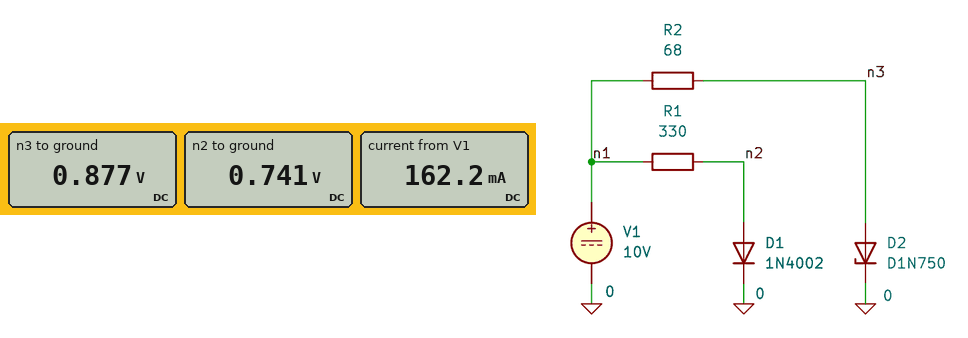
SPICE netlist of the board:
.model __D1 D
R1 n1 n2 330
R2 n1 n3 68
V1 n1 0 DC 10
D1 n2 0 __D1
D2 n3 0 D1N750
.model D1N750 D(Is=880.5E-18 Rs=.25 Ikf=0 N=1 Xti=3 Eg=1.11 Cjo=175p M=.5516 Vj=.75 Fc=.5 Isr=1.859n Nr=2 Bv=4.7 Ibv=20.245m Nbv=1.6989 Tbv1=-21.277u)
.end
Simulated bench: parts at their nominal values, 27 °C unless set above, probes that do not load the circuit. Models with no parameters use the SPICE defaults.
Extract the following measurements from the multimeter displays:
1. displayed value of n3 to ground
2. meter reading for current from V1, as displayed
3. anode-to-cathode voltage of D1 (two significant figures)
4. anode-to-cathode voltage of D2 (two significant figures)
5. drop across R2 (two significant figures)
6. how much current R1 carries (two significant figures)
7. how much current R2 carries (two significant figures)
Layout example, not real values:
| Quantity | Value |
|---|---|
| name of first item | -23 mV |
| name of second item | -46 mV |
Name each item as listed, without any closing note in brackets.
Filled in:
| Quantity | Value |
|---|---|
| displayed value of n3 to ground | 0.877 V |
| meter reading for current from V1, as displayed | 162.2 mA |
| anode-to-cathode voltage of D1 | 740 mV |
| anode-to-cathode voltage of D2 | 880 mV |
| drop across R2 | 9.1 V |
| how much current R1 carries | 28 mA |
| how much current R2 carries | 130 mA |
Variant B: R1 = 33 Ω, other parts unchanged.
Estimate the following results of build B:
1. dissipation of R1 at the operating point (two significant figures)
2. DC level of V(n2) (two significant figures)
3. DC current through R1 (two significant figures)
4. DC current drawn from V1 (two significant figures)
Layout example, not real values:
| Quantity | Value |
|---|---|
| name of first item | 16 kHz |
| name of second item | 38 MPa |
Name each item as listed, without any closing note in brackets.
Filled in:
| Quantity | Value |
|---|---|
| dissipation of R1 at the operating point | 2.6 W |
| DC level of V(n2) | 800 mV |
| DC current through R1 | 280 mA |
| DC current drawn from V1 | 410 mA |
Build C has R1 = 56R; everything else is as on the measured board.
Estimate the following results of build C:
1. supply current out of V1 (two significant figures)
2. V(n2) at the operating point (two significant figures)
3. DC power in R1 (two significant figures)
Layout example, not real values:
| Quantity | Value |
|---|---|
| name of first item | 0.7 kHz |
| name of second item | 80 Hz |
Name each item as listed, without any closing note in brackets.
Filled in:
| Quantity | Value |
|---|---|
| supply current out of V1 | 300 mA |
| V(n2) at the operating point | 790 mV |
| DC power in R1 | 1.5 W |
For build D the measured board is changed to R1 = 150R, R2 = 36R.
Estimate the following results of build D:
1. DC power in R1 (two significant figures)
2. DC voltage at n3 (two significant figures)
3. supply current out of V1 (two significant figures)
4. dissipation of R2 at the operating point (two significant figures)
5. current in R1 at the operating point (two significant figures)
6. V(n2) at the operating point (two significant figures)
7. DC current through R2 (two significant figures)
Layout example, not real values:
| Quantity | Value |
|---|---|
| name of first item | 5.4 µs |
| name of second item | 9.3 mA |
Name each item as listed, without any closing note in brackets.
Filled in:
| Quantity | Value |
|---|---|
| DC power in R1 | 570 mW |
| DC voltage at n3 | 920 mV |
| supply current out of V1 | 310 mA |
| dissipation of R2 at the operating point | 2.3 W |
| current in R1 at the operating point | 62 mA |
| V(n2) at the operating point | 760 mV |
| DC current through R2 | 250 mA |
